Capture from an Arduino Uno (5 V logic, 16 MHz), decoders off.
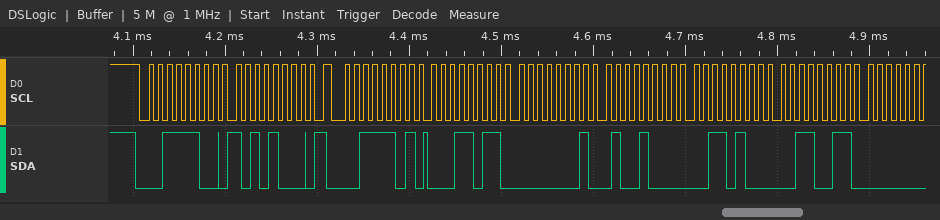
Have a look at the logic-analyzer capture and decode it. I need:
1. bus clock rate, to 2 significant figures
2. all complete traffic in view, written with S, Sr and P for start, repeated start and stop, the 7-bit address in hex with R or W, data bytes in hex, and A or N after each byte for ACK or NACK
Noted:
100 kHz
S 1EW A A8 A Sr 1ER A 1B A 01 A 48 A 34 A 33 A
